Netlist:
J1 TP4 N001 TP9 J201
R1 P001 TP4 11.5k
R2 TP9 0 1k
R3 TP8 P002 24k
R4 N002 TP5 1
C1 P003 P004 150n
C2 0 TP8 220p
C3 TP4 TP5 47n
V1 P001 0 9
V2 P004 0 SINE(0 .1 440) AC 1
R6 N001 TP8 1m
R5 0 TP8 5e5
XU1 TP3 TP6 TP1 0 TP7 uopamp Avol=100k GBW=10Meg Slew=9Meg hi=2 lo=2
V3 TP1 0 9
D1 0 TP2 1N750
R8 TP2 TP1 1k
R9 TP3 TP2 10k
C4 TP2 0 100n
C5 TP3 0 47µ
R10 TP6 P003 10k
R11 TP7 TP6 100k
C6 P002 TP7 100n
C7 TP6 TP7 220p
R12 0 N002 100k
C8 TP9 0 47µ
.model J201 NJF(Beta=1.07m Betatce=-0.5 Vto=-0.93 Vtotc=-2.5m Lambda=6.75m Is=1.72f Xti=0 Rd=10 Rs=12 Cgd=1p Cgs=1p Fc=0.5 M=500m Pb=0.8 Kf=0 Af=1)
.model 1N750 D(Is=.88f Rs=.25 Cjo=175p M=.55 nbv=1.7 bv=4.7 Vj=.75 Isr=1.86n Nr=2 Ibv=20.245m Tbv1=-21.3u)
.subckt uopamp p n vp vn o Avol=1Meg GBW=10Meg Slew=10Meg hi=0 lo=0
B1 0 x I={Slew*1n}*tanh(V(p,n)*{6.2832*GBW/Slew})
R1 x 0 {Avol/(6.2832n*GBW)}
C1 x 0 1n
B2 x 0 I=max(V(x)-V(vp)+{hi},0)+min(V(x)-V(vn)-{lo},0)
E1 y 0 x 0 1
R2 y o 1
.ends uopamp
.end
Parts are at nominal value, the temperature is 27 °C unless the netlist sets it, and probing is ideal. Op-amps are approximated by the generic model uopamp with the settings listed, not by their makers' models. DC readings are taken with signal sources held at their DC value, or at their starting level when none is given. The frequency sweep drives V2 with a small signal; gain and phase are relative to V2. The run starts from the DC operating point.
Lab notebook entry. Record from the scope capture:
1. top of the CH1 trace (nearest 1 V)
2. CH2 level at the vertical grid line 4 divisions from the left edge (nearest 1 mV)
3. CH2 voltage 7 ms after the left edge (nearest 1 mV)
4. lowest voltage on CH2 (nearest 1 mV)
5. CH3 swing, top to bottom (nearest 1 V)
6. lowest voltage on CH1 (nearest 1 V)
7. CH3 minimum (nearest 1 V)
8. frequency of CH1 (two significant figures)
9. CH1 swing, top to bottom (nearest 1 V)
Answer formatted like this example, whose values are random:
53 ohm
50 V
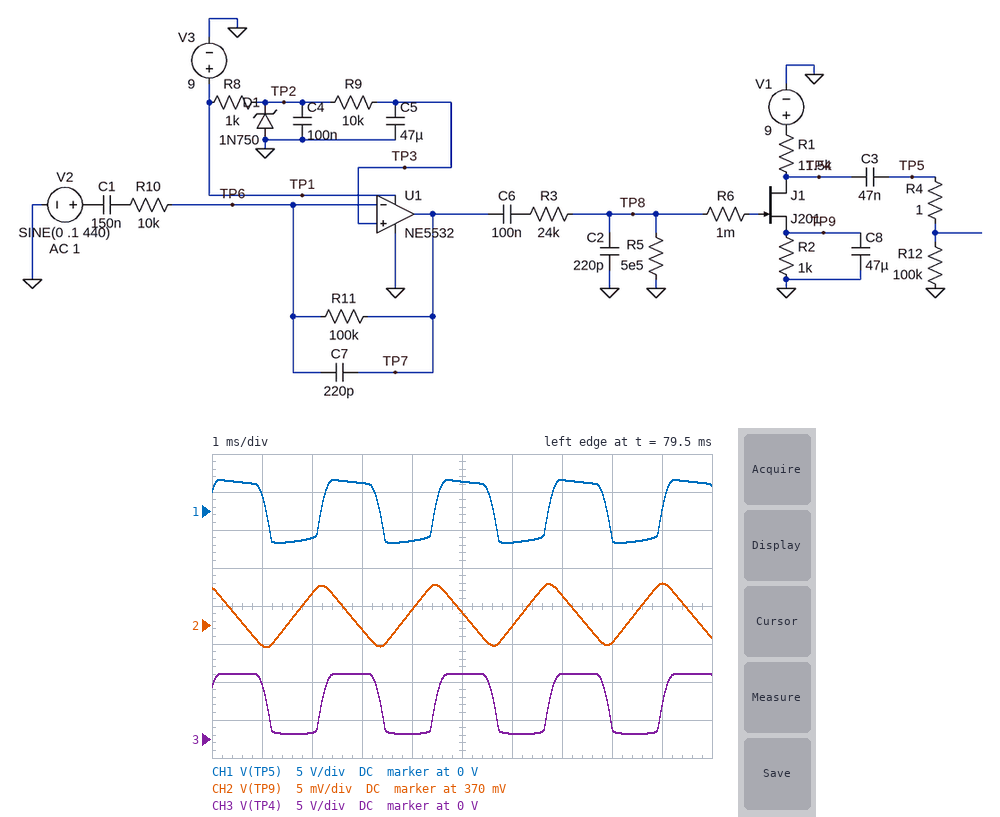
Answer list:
4 V
372 mV
374 mV
367 mV
8 V
-4 V
1 V
440 Hz
8 V
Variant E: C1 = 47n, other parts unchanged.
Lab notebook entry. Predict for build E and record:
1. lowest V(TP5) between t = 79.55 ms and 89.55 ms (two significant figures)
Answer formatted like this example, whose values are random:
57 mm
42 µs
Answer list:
-4.1 V
